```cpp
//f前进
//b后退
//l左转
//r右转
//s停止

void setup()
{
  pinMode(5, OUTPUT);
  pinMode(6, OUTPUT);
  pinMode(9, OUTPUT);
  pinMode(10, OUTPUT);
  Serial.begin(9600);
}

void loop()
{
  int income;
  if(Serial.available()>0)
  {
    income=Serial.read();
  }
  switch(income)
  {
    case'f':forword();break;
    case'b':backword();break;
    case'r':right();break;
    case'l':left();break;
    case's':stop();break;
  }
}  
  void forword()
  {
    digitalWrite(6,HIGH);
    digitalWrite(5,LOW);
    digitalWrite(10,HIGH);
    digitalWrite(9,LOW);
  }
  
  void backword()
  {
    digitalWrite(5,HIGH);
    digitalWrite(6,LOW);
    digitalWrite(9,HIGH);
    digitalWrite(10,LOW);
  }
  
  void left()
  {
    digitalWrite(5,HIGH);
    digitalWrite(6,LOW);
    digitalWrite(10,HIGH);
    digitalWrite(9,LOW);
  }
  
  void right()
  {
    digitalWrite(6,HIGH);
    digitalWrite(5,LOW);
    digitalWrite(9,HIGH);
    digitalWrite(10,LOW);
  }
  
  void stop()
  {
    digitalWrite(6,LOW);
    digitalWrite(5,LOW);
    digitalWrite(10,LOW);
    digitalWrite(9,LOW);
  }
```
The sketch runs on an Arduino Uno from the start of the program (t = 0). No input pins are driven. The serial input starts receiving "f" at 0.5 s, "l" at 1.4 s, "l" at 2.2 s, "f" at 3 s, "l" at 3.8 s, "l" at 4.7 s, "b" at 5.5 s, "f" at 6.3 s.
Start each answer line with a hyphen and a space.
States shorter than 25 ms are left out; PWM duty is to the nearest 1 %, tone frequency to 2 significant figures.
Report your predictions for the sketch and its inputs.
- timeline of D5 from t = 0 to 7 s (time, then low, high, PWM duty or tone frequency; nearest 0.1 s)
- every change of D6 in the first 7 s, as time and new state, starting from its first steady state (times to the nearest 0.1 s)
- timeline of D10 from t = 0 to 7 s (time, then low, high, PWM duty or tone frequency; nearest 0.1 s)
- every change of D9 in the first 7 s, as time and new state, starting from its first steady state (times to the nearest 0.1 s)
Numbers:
- 0 s low; 1.4 s high; 3 s low; 3.8 s high; 6.3 s low
- 0 s low; 0.5 s high; 1.4 s low; 3 s high; 3.8 s low; 6.3 s high
- 0 s low; 0.5 s high; 5.5 s low; 6.3 s high
- 0 s low; 5.5 s high; 6.3 s low
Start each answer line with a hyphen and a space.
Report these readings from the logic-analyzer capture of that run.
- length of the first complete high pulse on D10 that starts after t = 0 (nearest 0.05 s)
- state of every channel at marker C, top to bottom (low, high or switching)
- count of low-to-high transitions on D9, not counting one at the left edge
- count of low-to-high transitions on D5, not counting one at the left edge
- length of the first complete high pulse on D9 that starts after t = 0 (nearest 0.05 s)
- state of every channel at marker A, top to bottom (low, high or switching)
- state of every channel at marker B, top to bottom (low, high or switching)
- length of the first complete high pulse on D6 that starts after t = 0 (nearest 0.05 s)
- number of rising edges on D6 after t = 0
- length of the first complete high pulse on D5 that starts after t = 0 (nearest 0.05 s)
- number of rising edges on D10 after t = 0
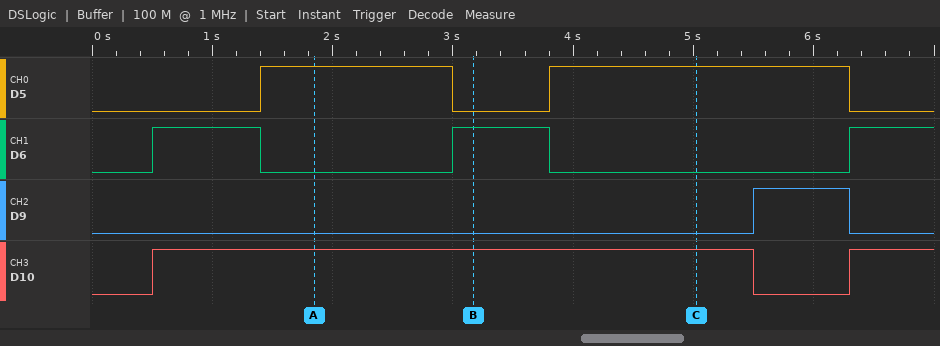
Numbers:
- 5.00 s
- D5 high, D6 low, D9 low, D10 high
- 1
- 2
- 0.80 s
- D5 high, D6 low, D9 low, D10 high
- D5 low, D6 high, D9 low, D10 high
- 0.90 s
- 3
- 1.60 s
- 2
